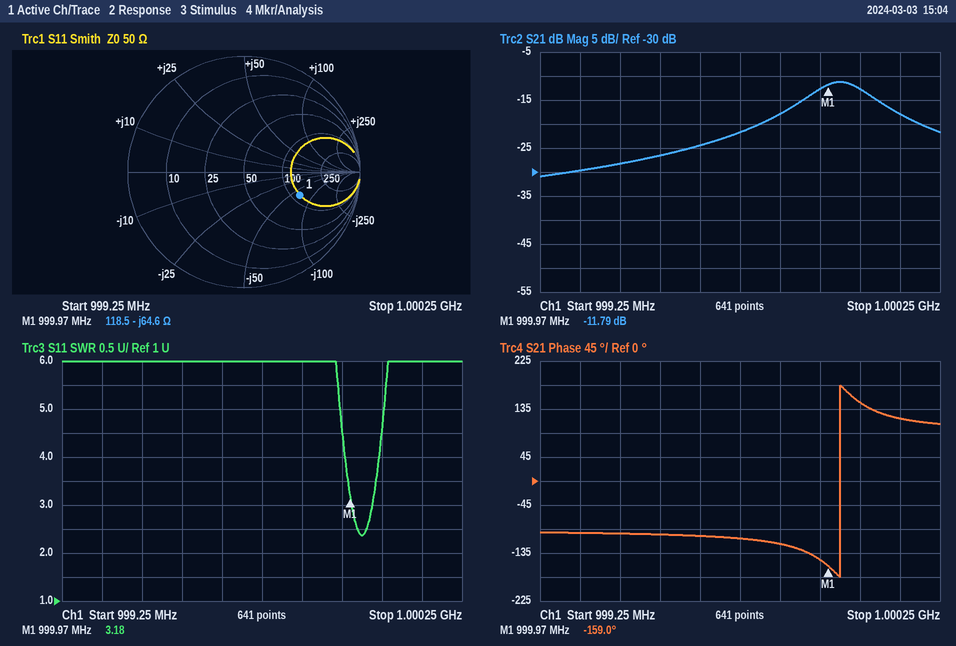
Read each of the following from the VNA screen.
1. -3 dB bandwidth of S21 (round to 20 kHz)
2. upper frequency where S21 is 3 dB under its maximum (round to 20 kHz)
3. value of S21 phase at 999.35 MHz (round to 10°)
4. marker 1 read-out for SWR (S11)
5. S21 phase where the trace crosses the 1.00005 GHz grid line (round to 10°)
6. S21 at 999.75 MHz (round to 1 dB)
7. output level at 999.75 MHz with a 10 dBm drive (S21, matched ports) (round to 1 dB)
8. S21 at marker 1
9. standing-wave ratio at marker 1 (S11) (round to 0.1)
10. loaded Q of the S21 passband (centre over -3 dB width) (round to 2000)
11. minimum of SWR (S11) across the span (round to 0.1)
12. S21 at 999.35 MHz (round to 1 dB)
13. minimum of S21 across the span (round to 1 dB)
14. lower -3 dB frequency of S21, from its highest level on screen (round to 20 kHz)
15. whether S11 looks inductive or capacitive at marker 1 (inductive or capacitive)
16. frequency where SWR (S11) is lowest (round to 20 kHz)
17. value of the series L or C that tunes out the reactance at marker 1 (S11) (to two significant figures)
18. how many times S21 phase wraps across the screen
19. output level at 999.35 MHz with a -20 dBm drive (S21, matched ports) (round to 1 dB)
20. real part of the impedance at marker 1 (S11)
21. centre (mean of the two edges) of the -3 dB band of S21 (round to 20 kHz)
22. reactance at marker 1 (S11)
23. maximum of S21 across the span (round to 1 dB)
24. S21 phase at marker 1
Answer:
160 kHz
1.00008 GHz
-100°
3.18
150°
-22 dB
-12 dBm
-11.79 dB
3.2
6000
2.4
-30 dB
-31 dB
999.92 MHz
capacitive
1.00000 GHz
10 nH
1
-50 dBm
118.5 Ω
1.00000 GHz
-64.6 Ω
-11 dB
-159.0°
